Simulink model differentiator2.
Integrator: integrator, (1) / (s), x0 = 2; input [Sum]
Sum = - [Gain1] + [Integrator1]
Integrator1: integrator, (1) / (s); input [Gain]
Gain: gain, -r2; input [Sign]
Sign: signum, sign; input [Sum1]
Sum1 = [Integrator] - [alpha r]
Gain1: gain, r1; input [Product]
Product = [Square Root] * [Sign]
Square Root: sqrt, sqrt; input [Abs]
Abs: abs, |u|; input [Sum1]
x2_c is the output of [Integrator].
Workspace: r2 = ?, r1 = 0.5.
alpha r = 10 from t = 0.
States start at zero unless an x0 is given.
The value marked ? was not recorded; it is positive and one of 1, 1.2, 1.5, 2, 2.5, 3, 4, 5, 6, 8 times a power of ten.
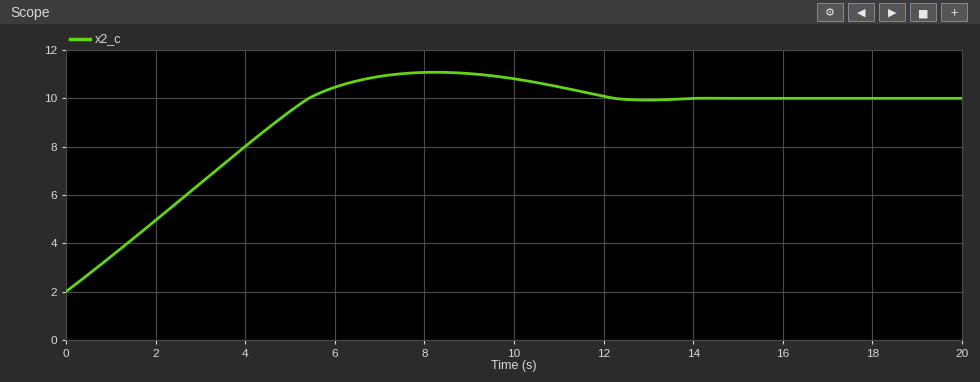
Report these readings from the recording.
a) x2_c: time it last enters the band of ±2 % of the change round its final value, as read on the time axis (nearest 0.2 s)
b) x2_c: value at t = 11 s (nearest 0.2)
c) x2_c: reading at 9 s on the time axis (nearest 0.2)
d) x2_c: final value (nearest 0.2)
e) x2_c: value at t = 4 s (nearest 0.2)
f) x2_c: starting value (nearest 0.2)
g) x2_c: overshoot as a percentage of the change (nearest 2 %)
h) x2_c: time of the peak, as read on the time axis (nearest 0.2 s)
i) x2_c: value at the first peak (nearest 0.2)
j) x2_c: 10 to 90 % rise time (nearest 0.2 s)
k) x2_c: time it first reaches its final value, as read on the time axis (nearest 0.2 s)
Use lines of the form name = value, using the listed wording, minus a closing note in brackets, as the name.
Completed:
x2_c: time it last enters the band of ±2 % of the change round its final value, as read on the time axis = 11.8 s
x2_c: value at t = 11 s = 10.4
x2_c: reading at 9 s on the time axis = 11.0
x2_c: final value = 10.0
x2_c: value at t = 4 s = 8.0
x2_c: starting value = 2.0
x2_c: overshoot as a percentage of the change = 14 %
x2_c: time of the peak, as read on the time axis = 8.2 s
x2_c: value at the first peak = 11.0
x2_c: 10 to 90 % rise time = 4.2 s
x2_c: time it first reaches its final value, as read on the time axis = 5.4 s
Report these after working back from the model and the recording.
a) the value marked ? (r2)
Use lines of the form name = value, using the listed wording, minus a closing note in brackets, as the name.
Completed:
the value marked ? = 0.2
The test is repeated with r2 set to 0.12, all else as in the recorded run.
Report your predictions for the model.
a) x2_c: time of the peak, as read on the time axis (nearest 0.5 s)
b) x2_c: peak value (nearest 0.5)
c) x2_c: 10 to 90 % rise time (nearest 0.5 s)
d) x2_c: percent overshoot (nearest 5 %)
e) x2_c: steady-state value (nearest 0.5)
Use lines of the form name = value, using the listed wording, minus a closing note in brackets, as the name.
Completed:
x2_c: time of the peak, as read on the time axis = 9.0 s
x2_c: peak value = 10.5
x2_c: 10 to 90 % rise time = 5.0 s
x2_c: percent overshoot = 10 %
x2_c: steady-state value = 10.0
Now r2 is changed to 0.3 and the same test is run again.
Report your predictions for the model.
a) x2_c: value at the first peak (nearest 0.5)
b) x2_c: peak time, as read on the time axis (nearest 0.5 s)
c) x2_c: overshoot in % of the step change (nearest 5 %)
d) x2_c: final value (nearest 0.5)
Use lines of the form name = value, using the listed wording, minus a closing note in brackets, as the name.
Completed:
x2_c: value at the first peak = 11.5
x2_c: peak time, as read on the time axis = 7.5 s
x2_c: overshoot in % of the step change = 20 %
x2_c: final value = 10.0
